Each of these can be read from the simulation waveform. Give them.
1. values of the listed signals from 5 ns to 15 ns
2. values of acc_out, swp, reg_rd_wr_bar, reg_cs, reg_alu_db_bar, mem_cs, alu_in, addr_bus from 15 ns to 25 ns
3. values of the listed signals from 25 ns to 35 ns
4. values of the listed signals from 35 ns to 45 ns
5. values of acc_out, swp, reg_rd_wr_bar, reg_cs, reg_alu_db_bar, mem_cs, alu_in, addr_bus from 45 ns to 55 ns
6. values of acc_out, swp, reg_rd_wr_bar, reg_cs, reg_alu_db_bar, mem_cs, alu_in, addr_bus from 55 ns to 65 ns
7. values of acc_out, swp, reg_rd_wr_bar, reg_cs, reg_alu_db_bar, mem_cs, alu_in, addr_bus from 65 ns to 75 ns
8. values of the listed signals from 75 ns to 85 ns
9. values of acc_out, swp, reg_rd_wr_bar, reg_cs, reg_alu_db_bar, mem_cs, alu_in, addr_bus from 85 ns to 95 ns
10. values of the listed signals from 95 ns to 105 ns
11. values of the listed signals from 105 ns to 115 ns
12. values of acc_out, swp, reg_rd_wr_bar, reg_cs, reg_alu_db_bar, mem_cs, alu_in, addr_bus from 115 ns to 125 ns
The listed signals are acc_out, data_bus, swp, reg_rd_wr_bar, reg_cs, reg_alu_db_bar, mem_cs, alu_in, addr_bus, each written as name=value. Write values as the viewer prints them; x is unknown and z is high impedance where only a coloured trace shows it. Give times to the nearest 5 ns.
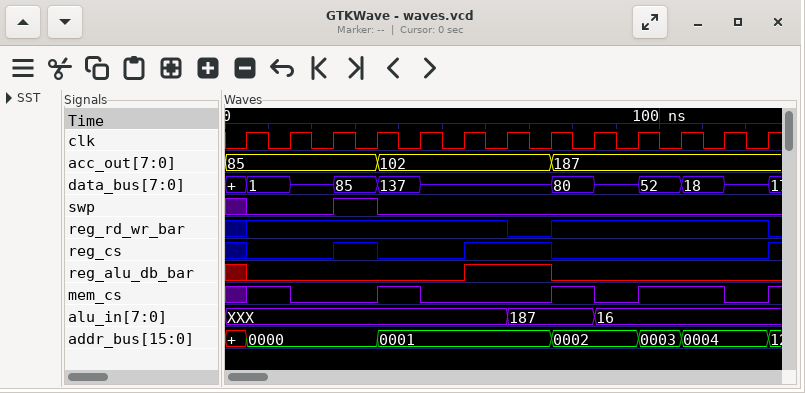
acc_out=85, data_bus=1, swp=0, reg_rd_wr_bar=1, reg_cs=0, reg_alu_db_bar=0, mem_cs=1, alu_in=XXX, addr_bus=0000
acc_out=85, swp=0, reg_rd_wr_bar=1, reg_cs=0, reg_alu_db_bar=0, mem_cs=0, alu_in=XXX, addr_bus=0000
acc_out=85, data_bus=85, swp=1, reg_rd_wr_bar=1, reg_cs=1, reg_alu_db_bar=0, mem_cs=0, alu_in=XXX, addr_bus=0000
acc_out=102, data_bus=137, swp=0, reg_rd_wr_bar=1, reg_cs=0, reg_alu_db_bar=0, mem_cs=1, alu_in=XXX, addr_bus=0001
acc_out=102, swp=0, reg_rd_wr_bar=1, reg_cs=0, reg_alu_db_bar=0, mem_cs=0, alu_in=XXX, addr_bus=0001
acc_out=102, swp=0, reg_rd_wr_bar=1, reg_cs=1, reg_alu_db_bar=1, mem_cs=0, alu_in=XXX, addr_bus=0001
acc_out=102, swp=0, reg_rd_wr_bar=0, reg_cs=1, reg_alu_db_bar=1, mem_cs=0, alu_in=187, addr_bus=0001
acc_out=187, data_bus=80, swp=0, reg_rd_wr_bar=1, reg_cs=0, reg_alu_db_bar=0, mem_cs=1, alu_in=187, addr_bus=0002
acc_out=187, swp=0, reg_rd_wr_bar=1, reg_cs=0, reg_alu_db_bar=0, mem_cs=0, alu_in=16, addr_bus=0002
acc_out=187, data_bus=52, swp=0, reg_rd_wr_bar=1, reg_cs=0, reg_alu_db_bar=0, mem_cs=1, alu_in=16, addr_bus=0003
acc_out=187, data_bus=18, swp=0, reg_rd_wr_bar=1, reg_cs=0, reg_alu_db_bar=0, mem_cs=1, alu_in=16, addr_bus=0004
acc_out=187, swp=0, reg_rd_wr_bar=1, reg_cs=0, reg_alu_db_bar=0, mem_cs=0, alu_in=16, addr_bus=0004
